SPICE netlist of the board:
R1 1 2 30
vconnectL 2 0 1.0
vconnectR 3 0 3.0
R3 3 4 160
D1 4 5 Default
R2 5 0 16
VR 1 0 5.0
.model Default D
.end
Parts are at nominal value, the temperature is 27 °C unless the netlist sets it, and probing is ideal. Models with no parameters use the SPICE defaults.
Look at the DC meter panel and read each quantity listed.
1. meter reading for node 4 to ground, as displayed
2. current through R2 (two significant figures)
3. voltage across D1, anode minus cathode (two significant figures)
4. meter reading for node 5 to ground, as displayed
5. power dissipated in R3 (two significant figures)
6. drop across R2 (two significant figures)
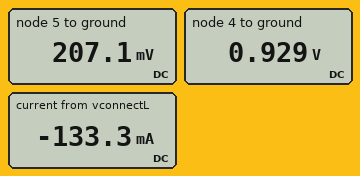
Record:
0.929 V
13 mA
720 mV
207.1 mV
27 mW
210 mV
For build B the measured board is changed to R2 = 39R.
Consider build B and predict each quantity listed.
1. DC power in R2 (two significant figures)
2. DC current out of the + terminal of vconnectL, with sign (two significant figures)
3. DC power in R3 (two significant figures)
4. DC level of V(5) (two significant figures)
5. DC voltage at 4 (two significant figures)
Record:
5.1 mW
-130 mA
21 mW
450 mV
1.2 V
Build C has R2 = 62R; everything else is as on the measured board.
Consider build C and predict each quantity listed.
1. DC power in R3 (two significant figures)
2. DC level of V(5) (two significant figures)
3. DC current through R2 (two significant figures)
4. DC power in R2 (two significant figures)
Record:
17 mW
640 mV
10 mA
6.6 mW
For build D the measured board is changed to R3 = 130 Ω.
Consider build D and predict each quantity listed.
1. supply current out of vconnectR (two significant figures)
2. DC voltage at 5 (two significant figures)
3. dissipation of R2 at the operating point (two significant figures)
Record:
16 mA
250 mV
3.9 mW
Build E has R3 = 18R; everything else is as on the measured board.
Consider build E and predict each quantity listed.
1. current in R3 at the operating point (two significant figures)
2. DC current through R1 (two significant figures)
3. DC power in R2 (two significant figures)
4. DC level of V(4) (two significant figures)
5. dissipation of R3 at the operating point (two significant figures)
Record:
66 mA
130 mA
69 mW
1.8 V
78 mW
